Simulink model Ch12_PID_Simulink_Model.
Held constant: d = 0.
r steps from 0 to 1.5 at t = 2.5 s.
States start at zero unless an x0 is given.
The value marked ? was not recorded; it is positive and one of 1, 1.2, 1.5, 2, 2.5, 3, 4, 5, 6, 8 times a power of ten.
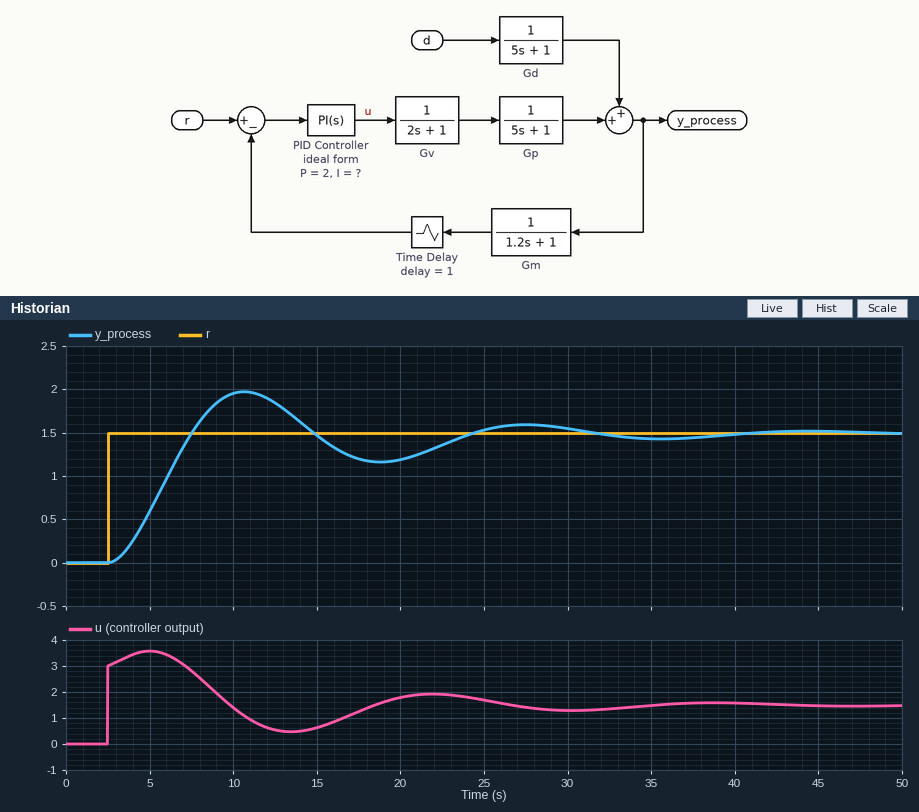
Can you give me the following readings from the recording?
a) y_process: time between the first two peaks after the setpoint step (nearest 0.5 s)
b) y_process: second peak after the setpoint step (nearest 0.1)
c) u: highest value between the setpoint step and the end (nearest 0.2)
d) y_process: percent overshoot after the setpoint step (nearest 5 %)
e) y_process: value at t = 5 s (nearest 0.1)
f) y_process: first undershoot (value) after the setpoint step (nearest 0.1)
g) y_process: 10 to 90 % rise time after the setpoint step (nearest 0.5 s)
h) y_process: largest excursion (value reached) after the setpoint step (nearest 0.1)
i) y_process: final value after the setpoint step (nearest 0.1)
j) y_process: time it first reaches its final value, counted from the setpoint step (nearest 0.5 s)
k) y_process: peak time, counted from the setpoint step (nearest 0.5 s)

17.0 s
1.6
3.6
30 %
0.6
1.2
3.5 s
2.0
1.5
5.0 s
8.0 s
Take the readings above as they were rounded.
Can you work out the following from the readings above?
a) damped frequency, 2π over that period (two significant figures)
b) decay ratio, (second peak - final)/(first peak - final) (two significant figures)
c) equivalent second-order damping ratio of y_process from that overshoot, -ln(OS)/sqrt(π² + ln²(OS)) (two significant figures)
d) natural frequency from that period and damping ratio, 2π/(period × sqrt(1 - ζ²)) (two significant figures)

0.37 rad/s
0.20
0.36
0.40 rad/s
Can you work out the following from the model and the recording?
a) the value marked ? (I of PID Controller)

0.1
